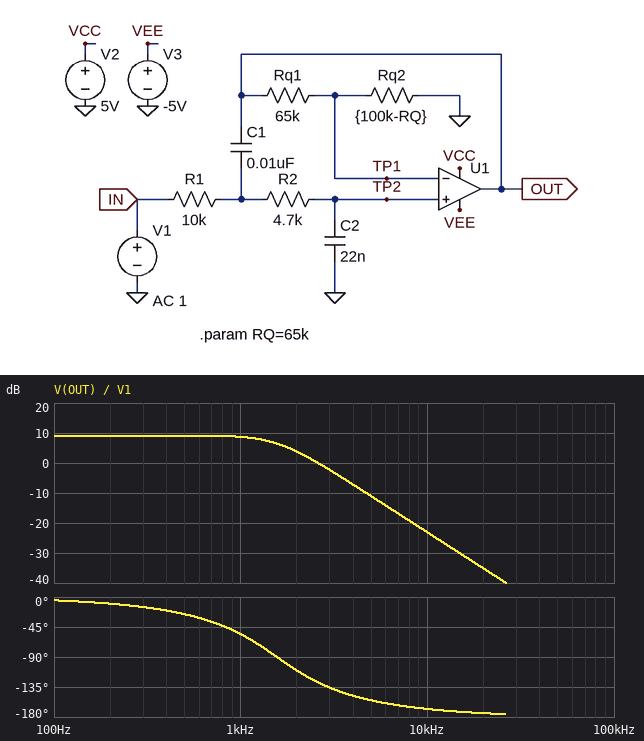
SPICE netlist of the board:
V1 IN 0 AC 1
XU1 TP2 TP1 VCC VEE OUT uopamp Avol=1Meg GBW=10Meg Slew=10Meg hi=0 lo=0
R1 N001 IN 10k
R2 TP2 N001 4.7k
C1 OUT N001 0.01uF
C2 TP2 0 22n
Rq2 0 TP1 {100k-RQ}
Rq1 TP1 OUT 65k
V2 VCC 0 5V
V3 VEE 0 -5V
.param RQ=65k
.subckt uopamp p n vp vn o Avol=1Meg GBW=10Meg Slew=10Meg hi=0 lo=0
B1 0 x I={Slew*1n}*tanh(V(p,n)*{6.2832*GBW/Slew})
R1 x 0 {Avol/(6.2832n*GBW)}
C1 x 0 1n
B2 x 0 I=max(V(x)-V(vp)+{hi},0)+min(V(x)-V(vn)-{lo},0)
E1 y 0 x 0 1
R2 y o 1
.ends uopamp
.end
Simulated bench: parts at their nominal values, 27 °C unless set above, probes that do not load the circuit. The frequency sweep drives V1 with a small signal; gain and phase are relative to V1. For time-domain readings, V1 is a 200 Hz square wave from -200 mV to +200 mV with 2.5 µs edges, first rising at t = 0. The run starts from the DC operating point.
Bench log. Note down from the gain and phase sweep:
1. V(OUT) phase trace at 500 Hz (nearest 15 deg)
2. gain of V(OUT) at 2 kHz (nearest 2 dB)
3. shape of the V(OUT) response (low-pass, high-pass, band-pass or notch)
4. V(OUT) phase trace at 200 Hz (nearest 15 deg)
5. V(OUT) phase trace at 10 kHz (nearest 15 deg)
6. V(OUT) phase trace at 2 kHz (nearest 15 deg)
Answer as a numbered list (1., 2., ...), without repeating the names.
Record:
1. -30 deg
2. 4 dB
3. low-pass
4. -15 deg
5. -165 deg
6. -105 deg
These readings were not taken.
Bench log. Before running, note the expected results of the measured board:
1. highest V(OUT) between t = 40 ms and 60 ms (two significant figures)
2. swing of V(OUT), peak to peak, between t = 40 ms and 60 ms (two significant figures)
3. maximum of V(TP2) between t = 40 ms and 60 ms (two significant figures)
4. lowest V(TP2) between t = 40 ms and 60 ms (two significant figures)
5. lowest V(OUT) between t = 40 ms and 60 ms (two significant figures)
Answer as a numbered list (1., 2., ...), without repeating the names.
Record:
1. 640 mV
2. 1.3 V
3. 220 mV
4. -220 mV
5. -640 mV
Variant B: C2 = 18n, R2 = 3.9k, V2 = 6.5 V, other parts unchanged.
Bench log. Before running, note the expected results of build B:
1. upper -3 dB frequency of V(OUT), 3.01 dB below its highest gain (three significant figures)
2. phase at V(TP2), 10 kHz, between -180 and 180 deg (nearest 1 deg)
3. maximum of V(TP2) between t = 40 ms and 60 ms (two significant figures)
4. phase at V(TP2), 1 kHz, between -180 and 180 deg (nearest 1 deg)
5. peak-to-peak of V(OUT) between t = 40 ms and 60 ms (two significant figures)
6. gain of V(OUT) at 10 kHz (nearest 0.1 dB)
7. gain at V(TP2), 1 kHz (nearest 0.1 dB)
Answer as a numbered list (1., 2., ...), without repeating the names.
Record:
1. 2.26 kHz
2. -171 deg
3. 310 mV
4. -29 deg
5. 1.8 V
6. -19.5 dB
7. 1.6 dB
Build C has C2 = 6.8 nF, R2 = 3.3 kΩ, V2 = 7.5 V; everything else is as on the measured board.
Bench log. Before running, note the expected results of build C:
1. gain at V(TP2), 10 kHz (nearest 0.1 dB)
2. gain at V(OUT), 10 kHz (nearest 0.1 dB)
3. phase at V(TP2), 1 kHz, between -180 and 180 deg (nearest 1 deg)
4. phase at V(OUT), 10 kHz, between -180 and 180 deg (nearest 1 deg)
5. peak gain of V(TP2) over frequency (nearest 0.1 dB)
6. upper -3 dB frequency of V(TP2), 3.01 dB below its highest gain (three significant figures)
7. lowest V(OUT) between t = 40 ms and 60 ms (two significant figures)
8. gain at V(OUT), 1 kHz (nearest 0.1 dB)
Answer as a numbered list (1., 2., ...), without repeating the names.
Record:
1. -19.9 dB
2. -10.8 dB
3. 33 deg
4. 143 deg
5. 0 dB
6. 2.15 kHz
7. -5.0 V
8. 8.4 dB
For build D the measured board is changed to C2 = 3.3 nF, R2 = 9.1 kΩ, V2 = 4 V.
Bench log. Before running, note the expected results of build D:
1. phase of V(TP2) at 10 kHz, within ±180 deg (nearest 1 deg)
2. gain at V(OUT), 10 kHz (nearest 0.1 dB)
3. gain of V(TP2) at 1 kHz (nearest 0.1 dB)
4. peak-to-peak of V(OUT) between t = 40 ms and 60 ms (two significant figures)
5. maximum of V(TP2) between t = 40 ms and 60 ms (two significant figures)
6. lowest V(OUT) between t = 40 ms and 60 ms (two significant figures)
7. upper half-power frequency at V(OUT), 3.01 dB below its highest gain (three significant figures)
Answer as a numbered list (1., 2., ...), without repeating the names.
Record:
1. 145 deg
2. -13.4 dB
3. -1.4 dB
4. 9.0 V
5. 3.6 V
6. -5.0 V
7. 1.60 kHz
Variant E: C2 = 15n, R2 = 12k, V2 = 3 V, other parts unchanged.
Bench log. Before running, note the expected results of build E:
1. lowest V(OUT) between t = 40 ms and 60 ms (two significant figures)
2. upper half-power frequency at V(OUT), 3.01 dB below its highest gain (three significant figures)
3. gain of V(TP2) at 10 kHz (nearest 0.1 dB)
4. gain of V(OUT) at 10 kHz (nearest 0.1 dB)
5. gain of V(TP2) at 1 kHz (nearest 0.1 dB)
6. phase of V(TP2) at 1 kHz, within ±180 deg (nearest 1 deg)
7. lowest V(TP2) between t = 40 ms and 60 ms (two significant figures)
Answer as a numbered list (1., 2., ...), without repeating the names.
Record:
1. -730 mV
2. 1.37 kHz
3. -37.0 dB
4. -27.9 dB
5. 0.4 dB
6. -72 deg
7. -250 mV
